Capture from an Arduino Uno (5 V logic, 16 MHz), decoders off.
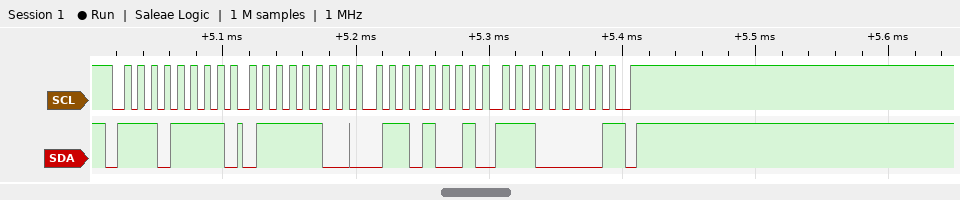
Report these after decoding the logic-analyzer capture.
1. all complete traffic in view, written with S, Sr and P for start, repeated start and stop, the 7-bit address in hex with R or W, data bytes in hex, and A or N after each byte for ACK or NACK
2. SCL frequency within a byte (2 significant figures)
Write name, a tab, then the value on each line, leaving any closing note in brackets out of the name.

all complete traffic in view, written with S, Sr and P for start, repeated start and stop, the 7-bit address in hex with R or W, data bytes in hex, and A or N after each byte for ACK or NACK	S 77R A 7C A 69 A E0 N P
SCL frequency within a byte	100 kHz
